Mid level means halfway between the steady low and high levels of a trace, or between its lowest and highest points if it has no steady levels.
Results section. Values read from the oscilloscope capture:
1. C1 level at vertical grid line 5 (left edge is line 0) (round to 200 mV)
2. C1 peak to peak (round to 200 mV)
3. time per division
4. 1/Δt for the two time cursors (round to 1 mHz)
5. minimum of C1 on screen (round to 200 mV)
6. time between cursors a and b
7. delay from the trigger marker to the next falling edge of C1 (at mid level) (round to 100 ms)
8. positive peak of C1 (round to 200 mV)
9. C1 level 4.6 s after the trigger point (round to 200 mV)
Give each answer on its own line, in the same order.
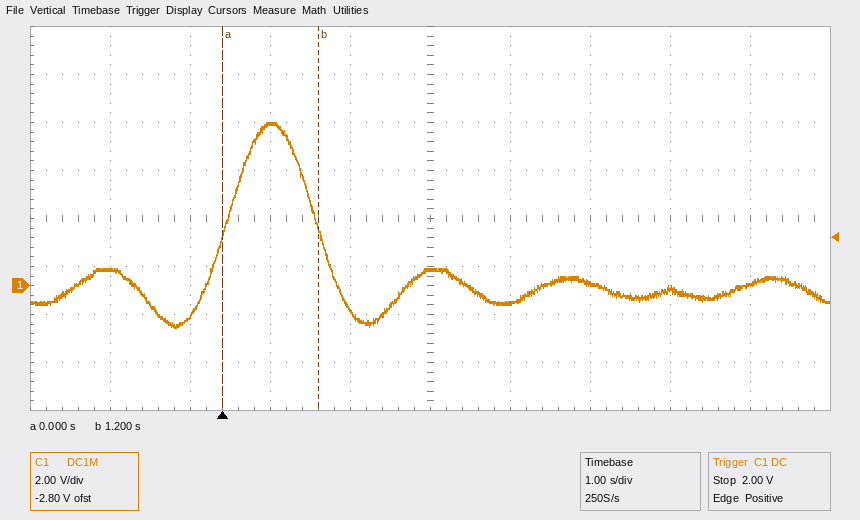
600 mV
8.6 V
1 s
833 mHz
-1.8 V
1.2 s
1.2 s
6.8 V
200 mV
